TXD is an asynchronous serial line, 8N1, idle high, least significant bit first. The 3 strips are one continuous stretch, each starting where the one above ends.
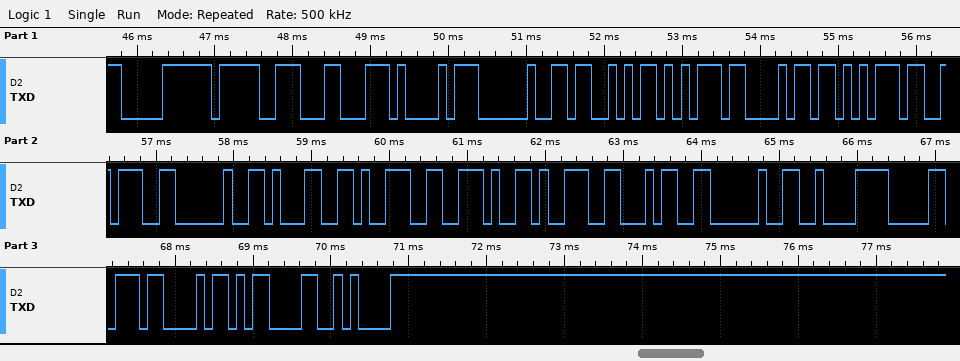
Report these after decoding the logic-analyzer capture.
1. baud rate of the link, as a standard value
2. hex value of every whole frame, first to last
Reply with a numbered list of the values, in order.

1. 9600 baud
2. F0 9F 8C A1 20 53 75 68 75 3A 20 31 39 2E 39 34 20 C2 B0 43 0D 0A
